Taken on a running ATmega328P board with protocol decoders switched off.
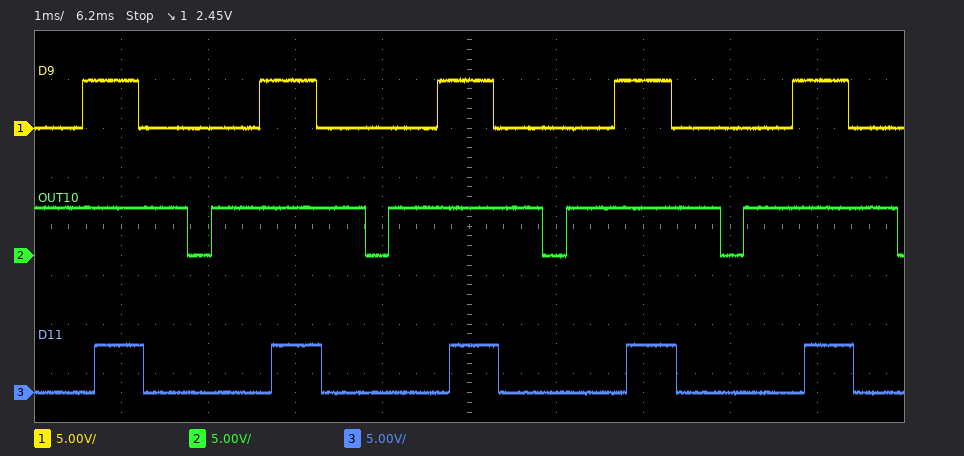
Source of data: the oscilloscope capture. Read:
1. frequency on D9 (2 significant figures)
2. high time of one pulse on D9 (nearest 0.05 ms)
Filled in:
490 Hz
0.65 ms
